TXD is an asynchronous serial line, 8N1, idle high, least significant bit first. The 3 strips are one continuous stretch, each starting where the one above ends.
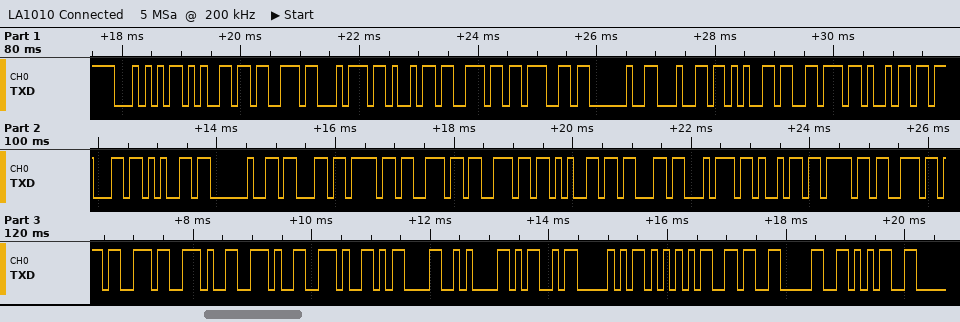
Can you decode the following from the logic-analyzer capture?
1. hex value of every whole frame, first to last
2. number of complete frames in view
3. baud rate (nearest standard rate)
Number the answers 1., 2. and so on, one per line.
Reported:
1. 0x54 0x65 0x73 0x74 0x69 0x6E 0x67 0x20 0x64 0x65 0x76 0x69 0x63 0x65 0x20 0x63 0x6F 0x6E 0x6E 0x65 0x63 0x74 0x69 0x6F 0x6E 0x73 0x2E 0x2E 0x2E 0x0D 0x0A 0x4D 0x50 0x55 0x36 0x30 0x35
2. 37
3. 9600 baud
